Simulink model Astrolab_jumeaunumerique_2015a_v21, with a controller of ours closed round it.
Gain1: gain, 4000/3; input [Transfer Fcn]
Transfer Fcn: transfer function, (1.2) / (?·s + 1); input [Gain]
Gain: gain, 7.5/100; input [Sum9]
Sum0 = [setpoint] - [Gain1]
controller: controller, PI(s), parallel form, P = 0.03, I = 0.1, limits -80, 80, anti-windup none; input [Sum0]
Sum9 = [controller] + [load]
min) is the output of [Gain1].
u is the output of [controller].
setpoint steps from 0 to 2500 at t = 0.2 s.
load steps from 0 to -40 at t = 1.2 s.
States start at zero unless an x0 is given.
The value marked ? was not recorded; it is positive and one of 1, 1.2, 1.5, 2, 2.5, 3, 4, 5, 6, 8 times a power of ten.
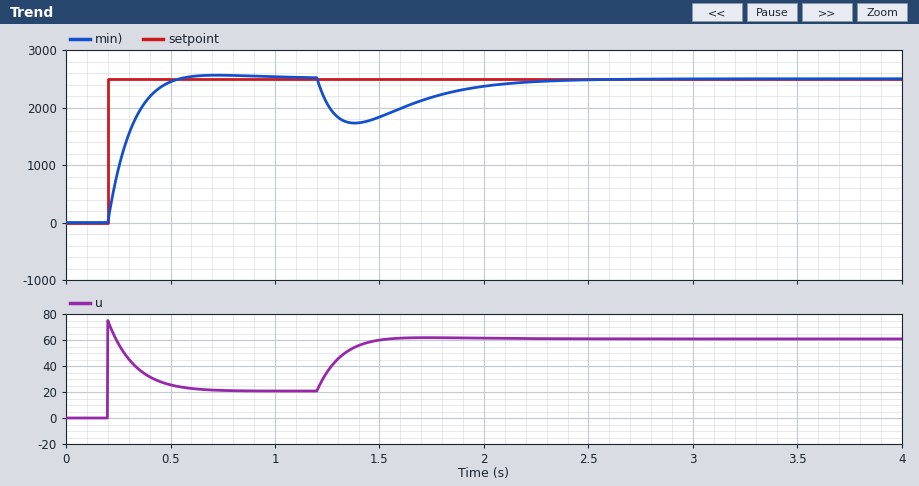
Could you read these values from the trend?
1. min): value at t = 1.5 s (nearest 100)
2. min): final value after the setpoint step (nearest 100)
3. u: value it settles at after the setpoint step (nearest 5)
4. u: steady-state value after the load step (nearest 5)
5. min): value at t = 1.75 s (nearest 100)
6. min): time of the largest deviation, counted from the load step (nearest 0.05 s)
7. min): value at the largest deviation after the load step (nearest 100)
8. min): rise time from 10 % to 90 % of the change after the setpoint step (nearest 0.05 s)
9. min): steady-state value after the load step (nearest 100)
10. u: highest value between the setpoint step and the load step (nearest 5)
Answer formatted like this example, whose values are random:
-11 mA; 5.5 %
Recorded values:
1800; 2500; 20; 60; 2200; 0.20 s; 1700; 0.20 s; 2500; 75
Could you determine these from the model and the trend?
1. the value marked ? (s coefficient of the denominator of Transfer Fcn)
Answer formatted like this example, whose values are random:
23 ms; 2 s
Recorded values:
0.4
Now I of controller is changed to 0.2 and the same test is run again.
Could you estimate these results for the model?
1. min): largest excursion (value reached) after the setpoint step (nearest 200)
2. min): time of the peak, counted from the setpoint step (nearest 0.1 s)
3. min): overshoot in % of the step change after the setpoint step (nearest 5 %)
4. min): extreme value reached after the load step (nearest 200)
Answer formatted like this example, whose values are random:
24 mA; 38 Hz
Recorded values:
2800; 0.3 s; 10 %; 1800
